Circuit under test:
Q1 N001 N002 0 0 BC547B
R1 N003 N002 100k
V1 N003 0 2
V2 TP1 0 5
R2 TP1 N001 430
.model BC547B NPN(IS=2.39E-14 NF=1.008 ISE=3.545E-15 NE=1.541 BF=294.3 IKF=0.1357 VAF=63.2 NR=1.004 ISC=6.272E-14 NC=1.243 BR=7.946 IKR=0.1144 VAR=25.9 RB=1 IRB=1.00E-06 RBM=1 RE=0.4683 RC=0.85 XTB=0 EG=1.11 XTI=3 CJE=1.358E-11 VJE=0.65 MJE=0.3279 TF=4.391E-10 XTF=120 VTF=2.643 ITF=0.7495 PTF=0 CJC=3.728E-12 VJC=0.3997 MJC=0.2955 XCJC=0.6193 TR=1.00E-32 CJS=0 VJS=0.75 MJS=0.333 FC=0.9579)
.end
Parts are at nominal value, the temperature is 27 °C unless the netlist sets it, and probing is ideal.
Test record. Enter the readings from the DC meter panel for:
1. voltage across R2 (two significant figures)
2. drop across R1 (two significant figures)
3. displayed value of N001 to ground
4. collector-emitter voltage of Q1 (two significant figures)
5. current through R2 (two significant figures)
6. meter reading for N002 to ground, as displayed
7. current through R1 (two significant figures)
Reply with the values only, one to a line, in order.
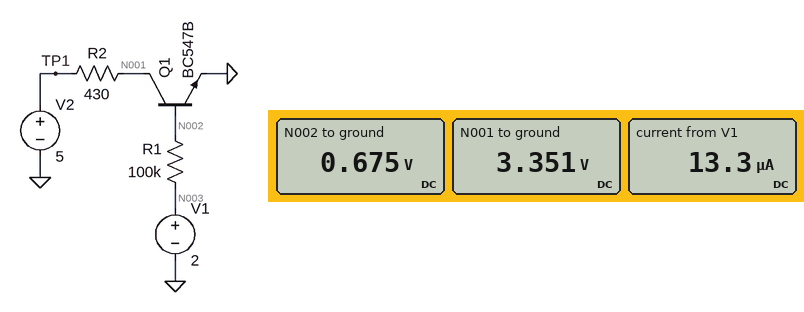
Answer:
1.6 V
1.3 V
3.351 V
3.4 V
3.8 mA
0.675 V
13 µA
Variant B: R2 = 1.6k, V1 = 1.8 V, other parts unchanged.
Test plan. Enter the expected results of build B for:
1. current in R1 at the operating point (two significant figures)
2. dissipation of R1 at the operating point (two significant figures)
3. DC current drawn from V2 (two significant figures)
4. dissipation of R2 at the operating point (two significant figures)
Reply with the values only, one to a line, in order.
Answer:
11 µA
13 µW
3.0 mA
14 mW
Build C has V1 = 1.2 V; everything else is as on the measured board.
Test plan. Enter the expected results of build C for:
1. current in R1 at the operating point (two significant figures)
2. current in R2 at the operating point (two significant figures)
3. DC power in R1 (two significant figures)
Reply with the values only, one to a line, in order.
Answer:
5.5 µA
1.6 mA
3.0 µW
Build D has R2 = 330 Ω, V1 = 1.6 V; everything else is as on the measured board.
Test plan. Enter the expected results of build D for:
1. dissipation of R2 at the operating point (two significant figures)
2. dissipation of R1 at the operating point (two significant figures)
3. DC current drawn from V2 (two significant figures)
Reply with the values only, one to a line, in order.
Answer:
2.5 mW
8.7 µW
2.8 mA
